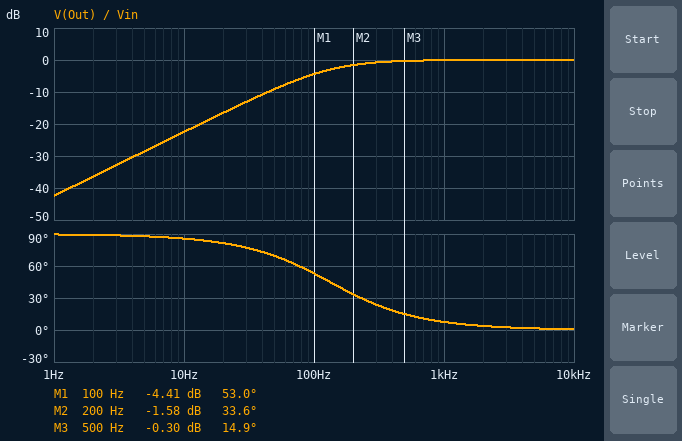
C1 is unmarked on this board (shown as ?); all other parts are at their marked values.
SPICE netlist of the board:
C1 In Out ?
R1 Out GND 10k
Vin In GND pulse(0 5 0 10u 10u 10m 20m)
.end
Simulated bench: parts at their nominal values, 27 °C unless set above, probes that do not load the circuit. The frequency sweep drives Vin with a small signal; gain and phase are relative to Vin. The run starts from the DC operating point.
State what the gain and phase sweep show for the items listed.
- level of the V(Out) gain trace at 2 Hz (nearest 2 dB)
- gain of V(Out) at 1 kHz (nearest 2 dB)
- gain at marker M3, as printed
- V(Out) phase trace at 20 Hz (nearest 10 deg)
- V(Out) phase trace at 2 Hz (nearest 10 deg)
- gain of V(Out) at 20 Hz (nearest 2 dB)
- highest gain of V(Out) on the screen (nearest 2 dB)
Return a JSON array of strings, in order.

["-36 dB", "0 dB", "-0.30 dB", "80 deg", "90 deg", "-16 dB", "0 dB"]
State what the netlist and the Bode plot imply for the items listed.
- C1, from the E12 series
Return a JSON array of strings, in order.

["120 nF"]
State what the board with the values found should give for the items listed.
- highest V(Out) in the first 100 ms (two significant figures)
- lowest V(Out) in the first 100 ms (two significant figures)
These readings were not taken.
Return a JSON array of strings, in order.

["5.0 V", "-5.0 V"]
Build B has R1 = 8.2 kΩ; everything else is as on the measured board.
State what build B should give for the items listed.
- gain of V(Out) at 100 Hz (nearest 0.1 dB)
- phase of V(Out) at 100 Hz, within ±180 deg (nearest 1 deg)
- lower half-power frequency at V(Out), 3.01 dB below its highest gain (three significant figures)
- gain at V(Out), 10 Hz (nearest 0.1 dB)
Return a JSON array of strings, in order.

["-5.6 dB", "58 deg", "162 Hz", "-24.2 dB"]
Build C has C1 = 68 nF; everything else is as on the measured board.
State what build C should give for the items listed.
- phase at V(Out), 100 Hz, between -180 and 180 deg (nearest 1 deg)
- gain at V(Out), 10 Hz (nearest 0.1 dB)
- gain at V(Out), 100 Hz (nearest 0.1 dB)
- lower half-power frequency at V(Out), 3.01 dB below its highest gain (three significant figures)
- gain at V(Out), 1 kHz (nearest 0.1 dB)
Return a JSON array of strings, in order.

["67 deg", "-27.4 dB", "-8.1 dB", "234 Hz", "-0.2 dB"]
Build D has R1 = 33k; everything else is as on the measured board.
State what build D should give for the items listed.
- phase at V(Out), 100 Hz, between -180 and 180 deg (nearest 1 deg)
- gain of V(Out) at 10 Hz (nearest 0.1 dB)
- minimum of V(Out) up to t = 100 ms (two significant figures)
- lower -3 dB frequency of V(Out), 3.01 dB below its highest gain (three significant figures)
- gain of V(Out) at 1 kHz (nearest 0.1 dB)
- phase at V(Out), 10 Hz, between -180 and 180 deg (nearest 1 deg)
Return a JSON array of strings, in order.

["22 deg", "-12.3 dB", "-4.6 V", "40.2 Hz", "0 dB", "76 deg"]
